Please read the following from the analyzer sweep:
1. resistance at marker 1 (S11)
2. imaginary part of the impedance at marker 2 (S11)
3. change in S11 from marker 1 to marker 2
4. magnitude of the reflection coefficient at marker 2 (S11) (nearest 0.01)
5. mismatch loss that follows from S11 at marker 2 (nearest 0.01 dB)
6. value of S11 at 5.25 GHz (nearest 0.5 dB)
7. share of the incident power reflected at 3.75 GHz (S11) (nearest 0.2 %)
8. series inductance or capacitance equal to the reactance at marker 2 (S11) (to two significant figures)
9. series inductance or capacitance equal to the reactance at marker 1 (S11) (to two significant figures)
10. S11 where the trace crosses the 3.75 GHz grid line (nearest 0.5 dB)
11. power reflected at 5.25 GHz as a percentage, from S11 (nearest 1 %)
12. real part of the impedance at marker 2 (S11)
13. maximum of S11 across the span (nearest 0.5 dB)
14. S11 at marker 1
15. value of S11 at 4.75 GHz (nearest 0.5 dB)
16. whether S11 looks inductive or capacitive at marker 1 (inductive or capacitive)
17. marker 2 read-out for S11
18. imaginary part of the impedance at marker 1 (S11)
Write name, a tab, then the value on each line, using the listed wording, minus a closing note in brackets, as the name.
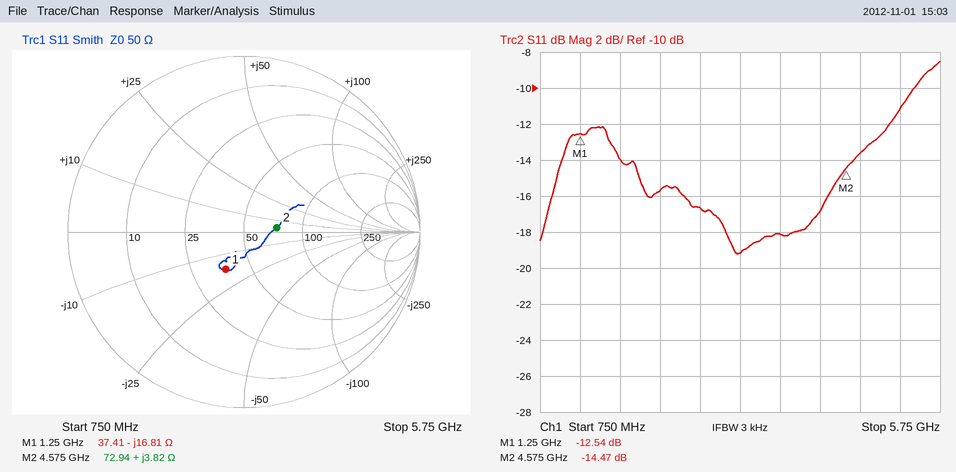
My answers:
resistance at marker 1	37.41 Ω
imaginary part of the impedance at marker 2	+3.82 Ω
change in S11 from marker 1 to marker 2	-1.93 dB
magnitude of the reflection coefficient at marker 2 (S11)	0.19
mismatch loss that follows from S11 at marker 2	0.16 dB
value of S11 at 5.25 GHz	-11.0 dB
share of the incident power reflected at 3.75 GHz (S11)	1.6 %
series inductance or capacitance equal to the reactance at marker 2 (S11)	130 pH
series inductance or capacitance equal to the reactance at marker 1 (S11)	7.6 pF
S11 where the trace crosses the 3.75 GHz grid line	-18.0 dB
power reflected at 5.25 GHz as a percentage, from S11	8 %
real part of the impedance at marker 2	72.94 Ω
maximum of S11 across the span	-8.5 dB
S11 at marker 1	-12.54 dB
value of S11 at 4.75 GHz	-13.5 dB
whether S11 looks inductive or capacitive at marker 1	capacitive
marker 2 read-out for S11	-14.47 dB
imaginary part of the impedance at marker 1	-16.81 Ω
